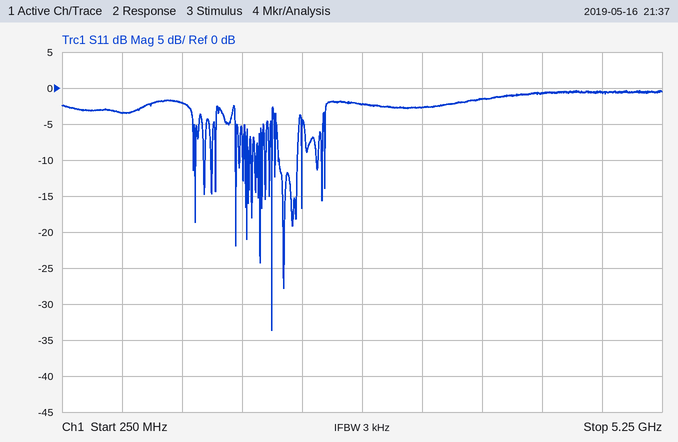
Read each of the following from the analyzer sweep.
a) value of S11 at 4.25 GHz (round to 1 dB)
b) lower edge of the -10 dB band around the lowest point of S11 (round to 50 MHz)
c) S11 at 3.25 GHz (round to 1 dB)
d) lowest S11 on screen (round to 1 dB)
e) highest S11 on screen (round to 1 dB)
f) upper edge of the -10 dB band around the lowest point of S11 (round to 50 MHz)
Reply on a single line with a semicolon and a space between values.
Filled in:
-1 dB; 2.00 GHz; -3 dB; -34 dB; 0 dB; 2.00 GHz
